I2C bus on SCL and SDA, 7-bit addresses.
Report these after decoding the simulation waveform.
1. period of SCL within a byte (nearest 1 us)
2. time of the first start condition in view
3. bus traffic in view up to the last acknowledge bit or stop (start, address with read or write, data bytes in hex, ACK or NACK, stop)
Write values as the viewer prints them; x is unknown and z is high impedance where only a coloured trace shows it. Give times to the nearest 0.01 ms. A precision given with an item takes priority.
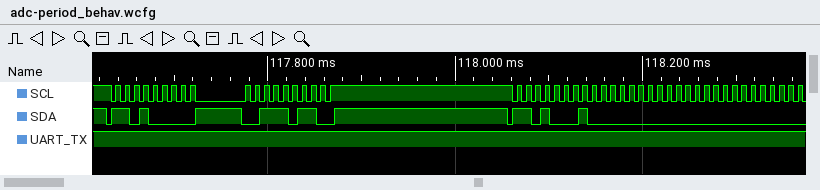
10 us
117.63 ms
start, address 68 write ACK, 3B ACK, stop, start, address 68 read ACK, 00 ACK, 00 ACK
